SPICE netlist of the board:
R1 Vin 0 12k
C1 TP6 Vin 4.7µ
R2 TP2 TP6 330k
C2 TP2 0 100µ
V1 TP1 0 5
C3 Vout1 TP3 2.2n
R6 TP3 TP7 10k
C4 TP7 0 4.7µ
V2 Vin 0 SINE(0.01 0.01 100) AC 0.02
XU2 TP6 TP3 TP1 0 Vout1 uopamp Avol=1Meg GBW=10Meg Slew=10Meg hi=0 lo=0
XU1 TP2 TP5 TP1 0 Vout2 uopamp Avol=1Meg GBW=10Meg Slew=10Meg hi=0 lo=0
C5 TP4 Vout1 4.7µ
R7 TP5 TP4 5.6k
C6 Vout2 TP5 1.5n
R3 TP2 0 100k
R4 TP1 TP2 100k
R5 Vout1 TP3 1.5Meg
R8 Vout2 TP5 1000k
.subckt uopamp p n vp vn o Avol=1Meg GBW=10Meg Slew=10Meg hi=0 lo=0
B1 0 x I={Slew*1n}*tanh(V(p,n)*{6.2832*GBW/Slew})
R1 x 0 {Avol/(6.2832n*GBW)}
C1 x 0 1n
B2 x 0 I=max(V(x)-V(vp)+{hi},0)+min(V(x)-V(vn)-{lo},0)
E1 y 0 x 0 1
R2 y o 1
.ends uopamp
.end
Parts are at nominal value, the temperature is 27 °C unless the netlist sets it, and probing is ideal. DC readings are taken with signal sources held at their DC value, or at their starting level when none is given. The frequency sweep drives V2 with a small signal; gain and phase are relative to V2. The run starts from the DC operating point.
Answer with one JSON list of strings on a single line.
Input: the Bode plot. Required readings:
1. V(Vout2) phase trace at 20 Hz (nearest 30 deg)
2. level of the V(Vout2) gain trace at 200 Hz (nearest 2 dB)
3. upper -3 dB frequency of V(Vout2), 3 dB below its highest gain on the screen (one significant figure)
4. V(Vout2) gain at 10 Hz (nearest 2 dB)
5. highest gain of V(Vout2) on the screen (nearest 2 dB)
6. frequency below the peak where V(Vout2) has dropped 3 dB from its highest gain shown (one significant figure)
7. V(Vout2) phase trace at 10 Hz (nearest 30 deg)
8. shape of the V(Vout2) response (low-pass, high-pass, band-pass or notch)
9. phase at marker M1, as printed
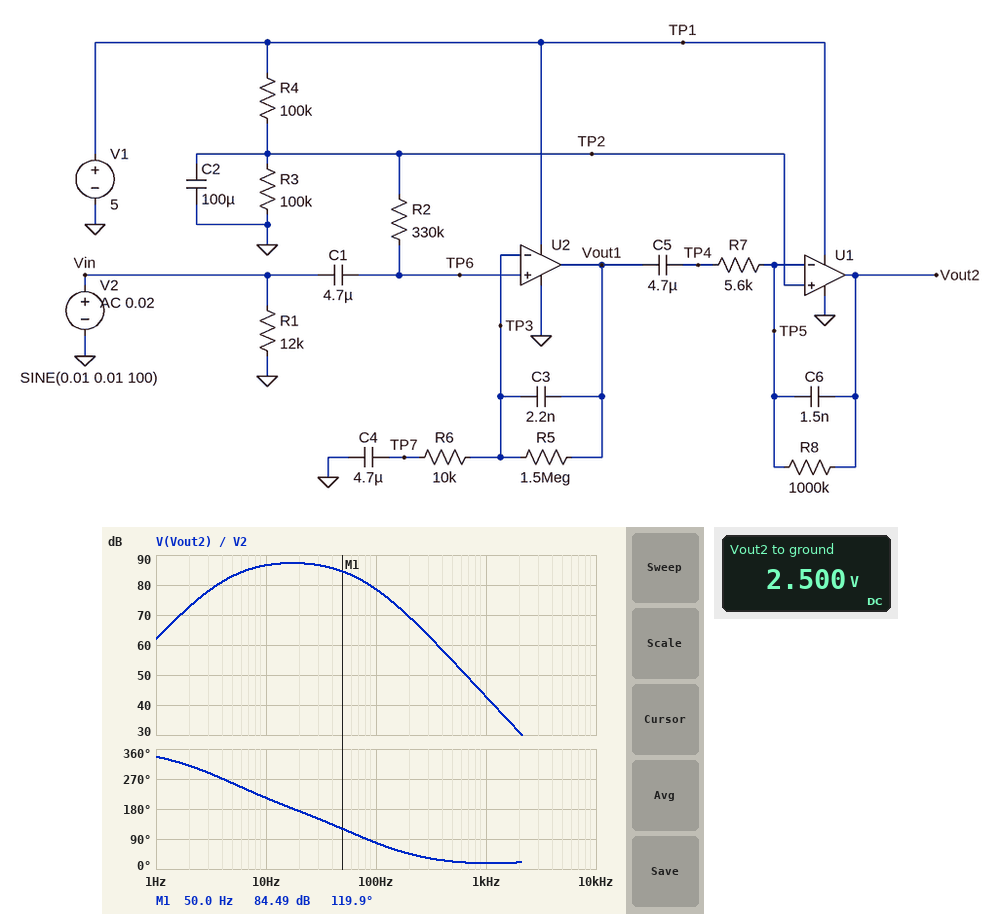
["180 deg", "70 dB", "50 Hz", "86 dB", "88 dB", "6 Hz", "210 deg", "band-pass", "119.9 deg"]
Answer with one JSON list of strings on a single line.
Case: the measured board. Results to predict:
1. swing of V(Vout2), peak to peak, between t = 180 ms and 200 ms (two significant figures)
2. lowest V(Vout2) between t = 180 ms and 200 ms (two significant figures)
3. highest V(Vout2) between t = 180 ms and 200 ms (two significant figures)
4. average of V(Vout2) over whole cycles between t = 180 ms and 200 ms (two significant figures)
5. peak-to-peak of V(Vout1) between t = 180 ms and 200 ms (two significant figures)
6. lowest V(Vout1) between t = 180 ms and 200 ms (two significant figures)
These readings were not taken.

["5.0 V", "-10 mV", "5.0 V", "2.5 V", "1.3 V", "1.8 V"]
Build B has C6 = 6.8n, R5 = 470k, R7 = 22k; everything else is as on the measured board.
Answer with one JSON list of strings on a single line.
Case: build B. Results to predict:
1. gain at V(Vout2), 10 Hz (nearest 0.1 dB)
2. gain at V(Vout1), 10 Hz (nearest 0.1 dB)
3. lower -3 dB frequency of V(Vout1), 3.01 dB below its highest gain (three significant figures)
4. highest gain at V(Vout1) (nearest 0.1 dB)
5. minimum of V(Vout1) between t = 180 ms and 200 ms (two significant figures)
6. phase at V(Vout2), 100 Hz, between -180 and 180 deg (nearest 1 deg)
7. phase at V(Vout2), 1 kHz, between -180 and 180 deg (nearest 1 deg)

["65.5 dB", "33.1 dB", "3.25 Hz", "33.4 dB", "2.1 V", "74 deg", "18 deg"]
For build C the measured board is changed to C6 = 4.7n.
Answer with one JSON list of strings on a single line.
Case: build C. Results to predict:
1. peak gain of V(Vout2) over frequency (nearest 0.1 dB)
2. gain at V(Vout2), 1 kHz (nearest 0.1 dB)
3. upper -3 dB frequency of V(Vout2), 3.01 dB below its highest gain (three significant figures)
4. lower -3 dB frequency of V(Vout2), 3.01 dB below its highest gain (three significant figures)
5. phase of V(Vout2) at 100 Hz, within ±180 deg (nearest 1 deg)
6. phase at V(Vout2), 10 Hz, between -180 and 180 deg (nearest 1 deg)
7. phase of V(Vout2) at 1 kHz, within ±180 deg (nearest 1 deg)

["86.6 dB", "32.9 dB", "34.4 Hz", "5.48 Hz", "51 deg", "-158 deg", "13 deg"]
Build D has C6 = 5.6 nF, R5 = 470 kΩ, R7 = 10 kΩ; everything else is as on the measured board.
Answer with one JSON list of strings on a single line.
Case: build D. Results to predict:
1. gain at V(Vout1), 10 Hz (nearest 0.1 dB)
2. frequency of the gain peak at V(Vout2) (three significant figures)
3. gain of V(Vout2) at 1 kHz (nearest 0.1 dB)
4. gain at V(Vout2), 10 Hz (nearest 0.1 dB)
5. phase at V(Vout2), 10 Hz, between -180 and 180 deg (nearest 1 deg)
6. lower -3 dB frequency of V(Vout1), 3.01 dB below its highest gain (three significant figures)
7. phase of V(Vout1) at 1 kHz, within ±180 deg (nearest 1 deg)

["33.1 dB", "11.8 Hz", "26.4 dB", "72.2 dB", "-165 deg", "3.25 Hz", "-73 deg"]
